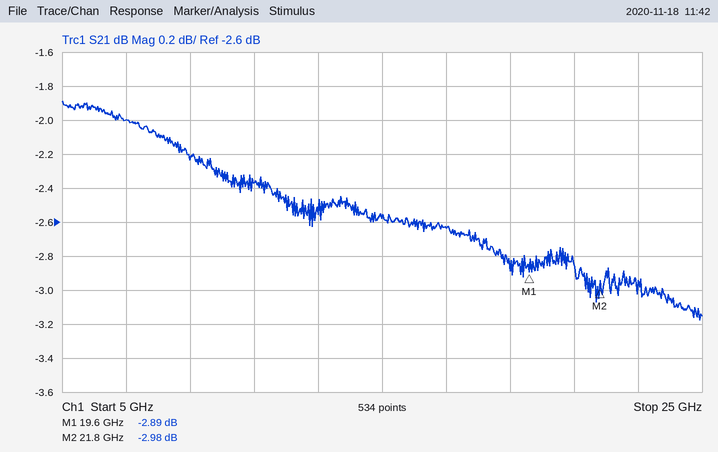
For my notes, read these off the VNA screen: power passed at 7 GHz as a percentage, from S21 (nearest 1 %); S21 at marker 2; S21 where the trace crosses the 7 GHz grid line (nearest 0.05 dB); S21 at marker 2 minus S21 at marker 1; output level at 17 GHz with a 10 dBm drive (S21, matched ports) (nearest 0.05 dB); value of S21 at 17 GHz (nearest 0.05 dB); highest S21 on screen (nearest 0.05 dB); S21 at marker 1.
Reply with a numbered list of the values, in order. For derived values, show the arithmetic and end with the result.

1. 10^(-2/10) ≈ 63 %
2. -2.98 dB
3. -2.00 dB
4. -2.98 − (-2.89) = -0.09 dB
5. 10 dBm + (-2.65 dB) = 7.35 dBm
6. -2.65 dB
7. -1.90 dB
8. -2.89 dB
